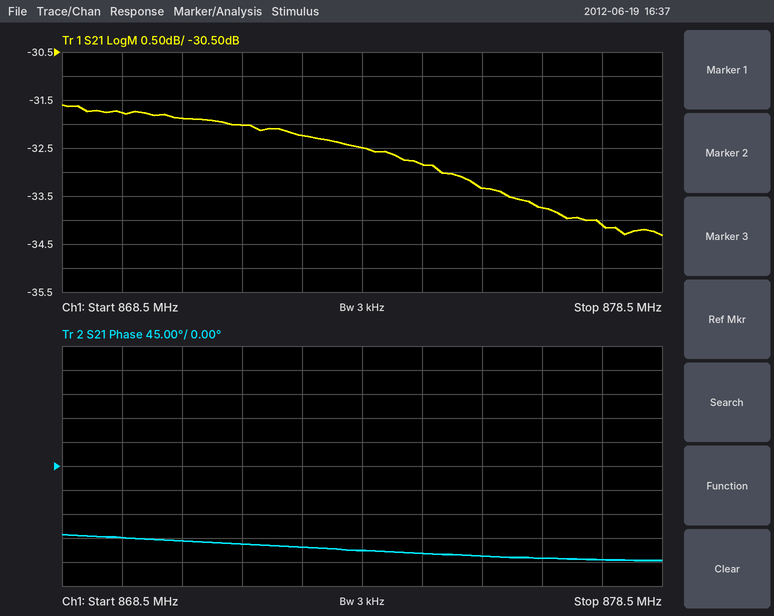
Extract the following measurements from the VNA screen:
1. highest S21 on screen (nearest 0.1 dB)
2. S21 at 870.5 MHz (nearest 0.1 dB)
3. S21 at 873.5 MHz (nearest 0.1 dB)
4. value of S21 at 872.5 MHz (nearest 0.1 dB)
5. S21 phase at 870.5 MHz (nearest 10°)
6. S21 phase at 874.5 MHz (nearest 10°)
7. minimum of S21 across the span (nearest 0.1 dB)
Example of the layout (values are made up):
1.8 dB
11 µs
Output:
-31.6 dB
-31.9 dB
-32.5 dB
-32.2 dB
-140°
-160°
-34.3 dB
